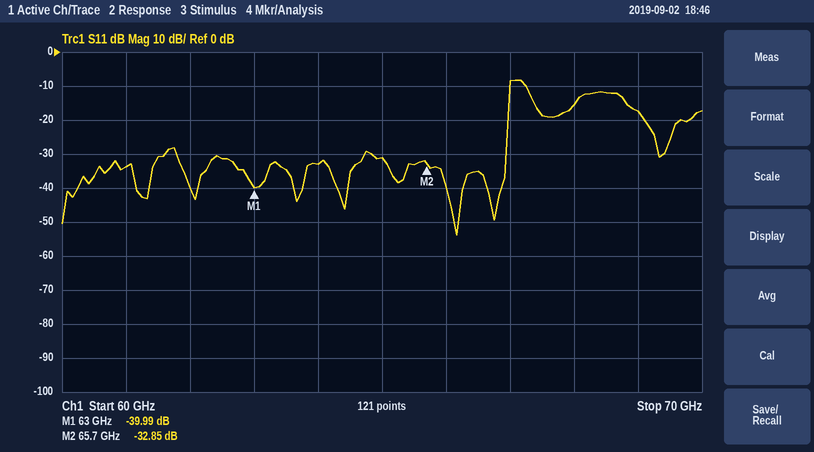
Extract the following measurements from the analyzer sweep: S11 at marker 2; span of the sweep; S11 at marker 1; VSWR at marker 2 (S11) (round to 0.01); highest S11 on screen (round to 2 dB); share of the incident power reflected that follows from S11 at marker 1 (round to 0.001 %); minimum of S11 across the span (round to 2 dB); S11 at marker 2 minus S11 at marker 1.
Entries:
-32.85 dB
10 GHz
-39.99 dB
1.05
-8 dB
0.010 %
-54 dB
7.14 dB
